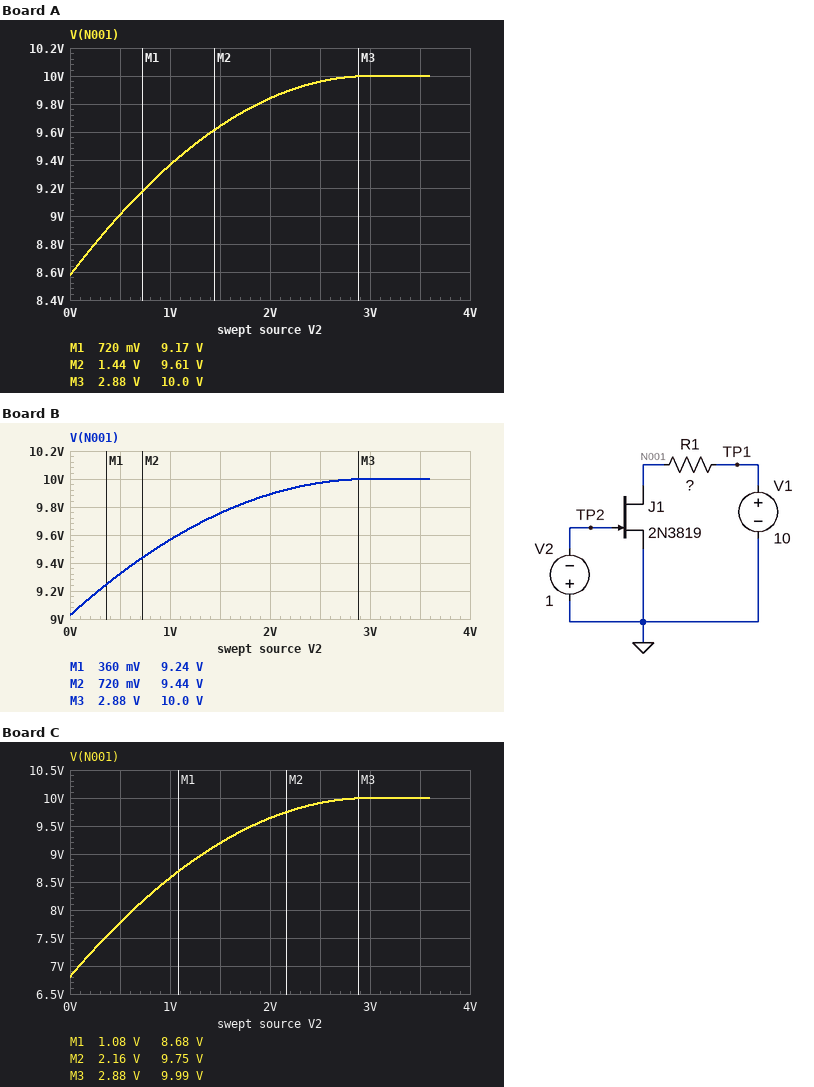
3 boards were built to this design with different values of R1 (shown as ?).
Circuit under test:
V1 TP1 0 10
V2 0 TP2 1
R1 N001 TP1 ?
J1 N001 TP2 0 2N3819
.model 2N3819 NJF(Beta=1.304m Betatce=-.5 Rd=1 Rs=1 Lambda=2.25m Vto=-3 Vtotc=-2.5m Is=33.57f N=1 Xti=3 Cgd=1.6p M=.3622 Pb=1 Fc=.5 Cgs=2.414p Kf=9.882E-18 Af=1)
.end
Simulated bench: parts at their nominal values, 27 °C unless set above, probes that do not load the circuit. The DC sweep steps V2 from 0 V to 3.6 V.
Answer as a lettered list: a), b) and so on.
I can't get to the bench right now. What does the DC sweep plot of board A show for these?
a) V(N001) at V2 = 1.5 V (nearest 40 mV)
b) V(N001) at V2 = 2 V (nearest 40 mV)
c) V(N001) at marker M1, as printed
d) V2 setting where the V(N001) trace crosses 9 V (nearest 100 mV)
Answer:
a) 9.64 V
b) 9.84 V
c) 9.17 V
d) 500 mV
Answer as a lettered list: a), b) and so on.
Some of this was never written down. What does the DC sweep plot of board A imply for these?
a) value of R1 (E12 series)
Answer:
a) 120 Ω
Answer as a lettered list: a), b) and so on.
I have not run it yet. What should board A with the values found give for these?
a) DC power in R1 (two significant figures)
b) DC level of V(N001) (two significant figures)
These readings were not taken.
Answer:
a) 3.4 mW
b) 9.4 V
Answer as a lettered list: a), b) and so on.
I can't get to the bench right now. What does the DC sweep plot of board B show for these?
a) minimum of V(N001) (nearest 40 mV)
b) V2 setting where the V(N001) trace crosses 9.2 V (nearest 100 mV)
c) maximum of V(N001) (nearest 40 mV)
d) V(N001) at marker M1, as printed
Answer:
a) 9.04 V
b) 300 mV
c) 10.00 V
d) 9.24 V
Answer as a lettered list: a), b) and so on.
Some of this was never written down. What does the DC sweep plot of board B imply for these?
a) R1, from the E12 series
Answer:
a) 82 Ω
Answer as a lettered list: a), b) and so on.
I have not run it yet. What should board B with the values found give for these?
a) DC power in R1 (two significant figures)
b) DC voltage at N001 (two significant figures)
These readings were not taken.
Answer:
a) 2.3 mW
b) 9.6 V
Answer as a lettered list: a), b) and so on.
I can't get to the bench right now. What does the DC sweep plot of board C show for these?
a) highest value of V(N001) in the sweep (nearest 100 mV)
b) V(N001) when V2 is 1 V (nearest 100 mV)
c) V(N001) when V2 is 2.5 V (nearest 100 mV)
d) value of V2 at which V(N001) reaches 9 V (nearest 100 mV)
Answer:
a) 10.0 V
b) 8.6 V
c) 9.9 V
d) 1.3 V
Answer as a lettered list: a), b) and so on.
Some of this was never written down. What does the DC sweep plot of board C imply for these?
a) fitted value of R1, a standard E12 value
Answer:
a) 270 Ω
